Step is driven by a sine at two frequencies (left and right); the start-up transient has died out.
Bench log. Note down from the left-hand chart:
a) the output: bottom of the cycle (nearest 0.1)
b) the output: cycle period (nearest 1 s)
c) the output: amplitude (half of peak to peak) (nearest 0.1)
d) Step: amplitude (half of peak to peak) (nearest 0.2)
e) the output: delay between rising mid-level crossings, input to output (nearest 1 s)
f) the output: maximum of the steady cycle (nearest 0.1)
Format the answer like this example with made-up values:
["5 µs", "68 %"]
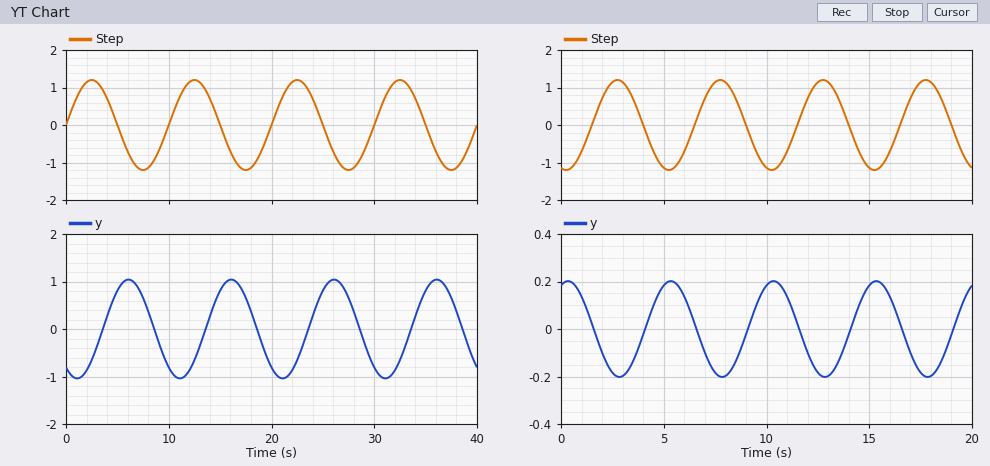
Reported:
["-1.0", "10 s", "1.0", "1.2", "4 s", "1.0"]
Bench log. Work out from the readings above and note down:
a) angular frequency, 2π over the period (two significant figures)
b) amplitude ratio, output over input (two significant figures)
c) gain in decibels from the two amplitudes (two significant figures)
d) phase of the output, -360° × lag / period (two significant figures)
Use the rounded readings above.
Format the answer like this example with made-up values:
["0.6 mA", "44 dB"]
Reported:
["0.63 rad/s", "0.83", "-1.6 dB", "-140°"]
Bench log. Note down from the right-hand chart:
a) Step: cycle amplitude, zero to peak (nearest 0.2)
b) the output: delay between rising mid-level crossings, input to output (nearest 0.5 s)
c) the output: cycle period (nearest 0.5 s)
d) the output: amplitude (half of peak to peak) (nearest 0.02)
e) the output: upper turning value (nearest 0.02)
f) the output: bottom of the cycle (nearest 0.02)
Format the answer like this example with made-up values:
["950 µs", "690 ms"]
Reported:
["1.2", "2.5 s", "5.0 s", "0.20", "0.20", "-0.20"]
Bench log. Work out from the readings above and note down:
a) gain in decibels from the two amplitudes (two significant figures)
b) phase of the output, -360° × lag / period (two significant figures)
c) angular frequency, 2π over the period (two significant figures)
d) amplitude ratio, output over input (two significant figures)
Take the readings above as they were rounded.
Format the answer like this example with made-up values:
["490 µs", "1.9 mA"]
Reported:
["-16 dB", "-180°", "1.3 rad/s", "0.17"]
